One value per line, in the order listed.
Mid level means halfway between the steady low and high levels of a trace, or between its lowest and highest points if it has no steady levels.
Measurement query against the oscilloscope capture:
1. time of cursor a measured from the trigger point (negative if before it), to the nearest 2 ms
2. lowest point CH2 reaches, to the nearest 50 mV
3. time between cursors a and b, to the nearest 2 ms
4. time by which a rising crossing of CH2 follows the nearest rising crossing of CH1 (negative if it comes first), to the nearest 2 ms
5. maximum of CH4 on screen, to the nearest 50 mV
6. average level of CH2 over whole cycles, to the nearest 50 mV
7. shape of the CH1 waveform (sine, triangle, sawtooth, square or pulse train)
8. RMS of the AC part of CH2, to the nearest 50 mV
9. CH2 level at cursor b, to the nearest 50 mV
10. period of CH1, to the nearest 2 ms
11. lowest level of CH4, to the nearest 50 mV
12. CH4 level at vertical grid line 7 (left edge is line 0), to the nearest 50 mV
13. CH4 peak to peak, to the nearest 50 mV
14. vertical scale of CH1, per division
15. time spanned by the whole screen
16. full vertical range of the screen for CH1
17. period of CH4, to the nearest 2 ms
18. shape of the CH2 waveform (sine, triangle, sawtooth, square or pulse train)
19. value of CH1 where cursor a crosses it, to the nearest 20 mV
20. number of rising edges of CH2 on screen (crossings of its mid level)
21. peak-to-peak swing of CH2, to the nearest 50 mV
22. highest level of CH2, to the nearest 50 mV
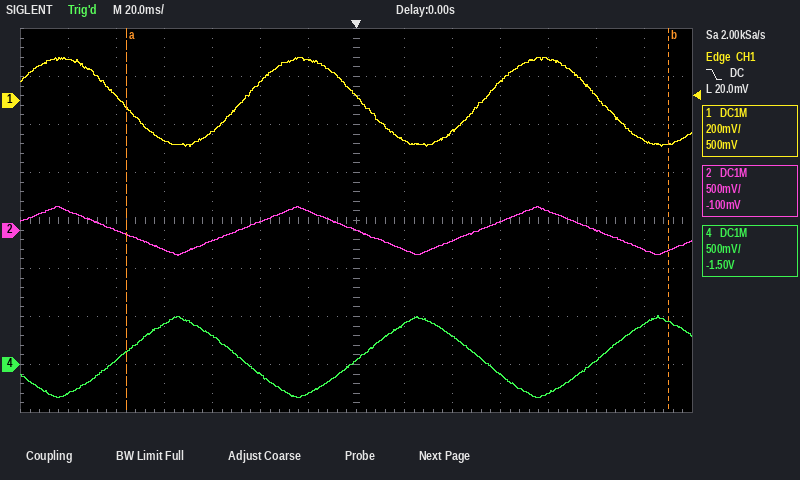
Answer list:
-96 ms
-250 mV
226 ms
-2 ms
500 mV
0 mV
sine
150 mV
-200 mV
100 ms
-350 mV
50 mV
850 mV
200 mV
280 ms
1.6 V
100 ms
triangle
-20 mV
2
500 mV
250 mV
